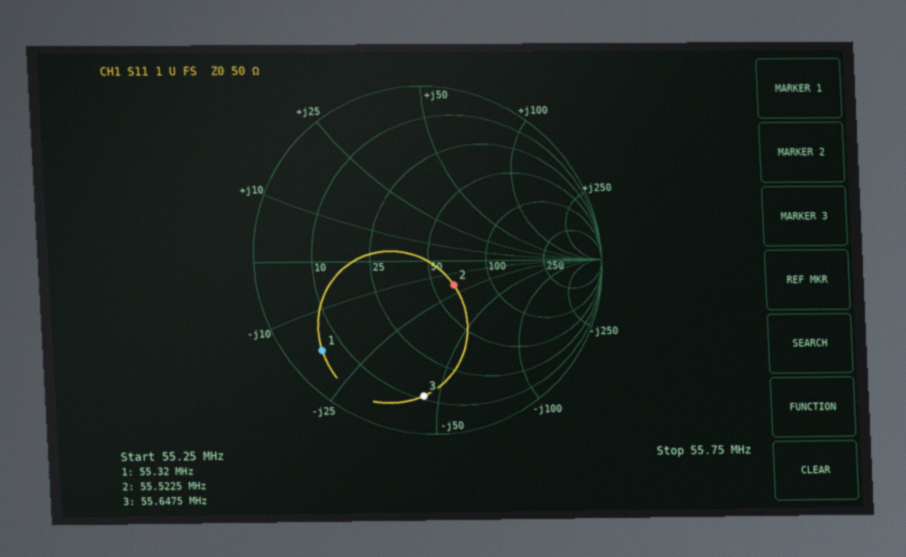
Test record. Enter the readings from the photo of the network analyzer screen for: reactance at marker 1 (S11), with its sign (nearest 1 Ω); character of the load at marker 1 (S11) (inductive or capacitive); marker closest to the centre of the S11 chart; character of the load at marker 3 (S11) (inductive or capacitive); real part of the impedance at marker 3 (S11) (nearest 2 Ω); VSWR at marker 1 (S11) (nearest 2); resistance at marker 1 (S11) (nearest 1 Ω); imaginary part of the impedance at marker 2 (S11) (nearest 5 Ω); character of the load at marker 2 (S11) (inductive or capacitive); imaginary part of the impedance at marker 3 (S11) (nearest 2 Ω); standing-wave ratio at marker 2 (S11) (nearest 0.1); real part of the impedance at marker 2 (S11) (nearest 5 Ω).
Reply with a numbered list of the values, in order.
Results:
1. -17 Ω
2. capacitive
3. marker 2
4. capacitive
5. 12 Ω
6. 10
7. 6 Ω
8. -20 Ω
9. capacitive
10. -44 Ω
11. 1.5
12. 65 Ω
